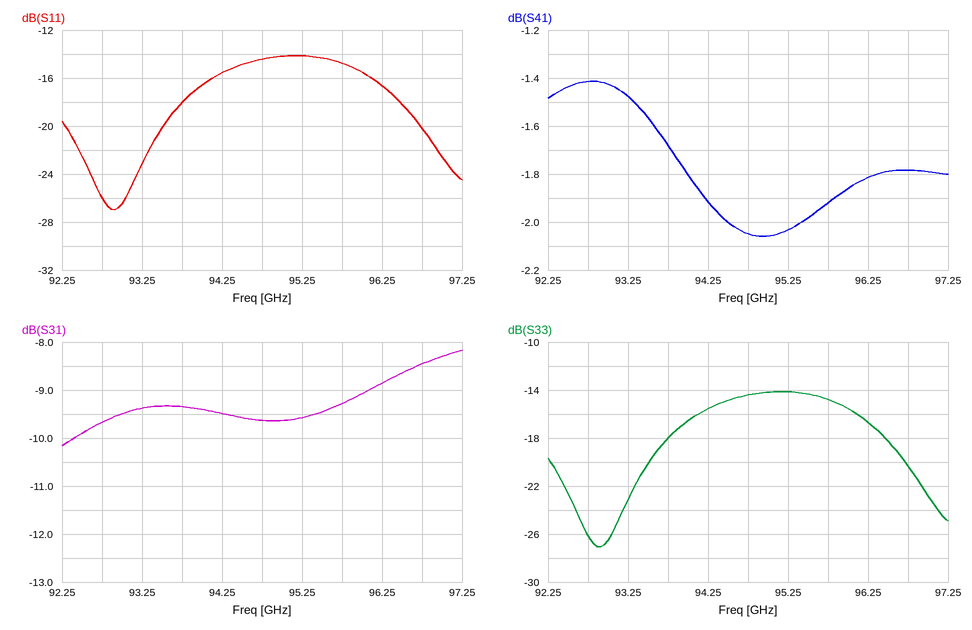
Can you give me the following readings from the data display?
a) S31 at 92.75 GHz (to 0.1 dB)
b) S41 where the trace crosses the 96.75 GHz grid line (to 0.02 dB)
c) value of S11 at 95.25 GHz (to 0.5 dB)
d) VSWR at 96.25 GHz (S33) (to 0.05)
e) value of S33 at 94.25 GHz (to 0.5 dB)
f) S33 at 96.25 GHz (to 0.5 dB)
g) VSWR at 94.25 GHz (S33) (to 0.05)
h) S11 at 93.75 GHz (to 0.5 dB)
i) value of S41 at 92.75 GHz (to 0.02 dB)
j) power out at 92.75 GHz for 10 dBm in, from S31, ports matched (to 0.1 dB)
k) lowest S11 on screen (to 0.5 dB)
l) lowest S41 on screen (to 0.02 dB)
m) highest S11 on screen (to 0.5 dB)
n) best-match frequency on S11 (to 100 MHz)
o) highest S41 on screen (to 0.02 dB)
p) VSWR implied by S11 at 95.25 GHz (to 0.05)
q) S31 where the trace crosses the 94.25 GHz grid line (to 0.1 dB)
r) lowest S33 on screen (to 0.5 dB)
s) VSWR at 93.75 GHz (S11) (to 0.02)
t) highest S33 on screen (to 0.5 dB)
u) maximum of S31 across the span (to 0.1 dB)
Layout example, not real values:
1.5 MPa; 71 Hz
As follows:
-9.7 dB; -1.78 dB; -14.0 dB; 1.35; -15.5 dB; -16.5 dB; 1.40; -18.0 dB; -1.42 dB; 0.3 dBm; -27.0 dB; -2.06 dB; -14.0 dB; 92.9 GHz; -1.42 dB; 1.50; -9.5 dB; -27.0 dB; 1.28; -14.0 dB; -8.2 dB
